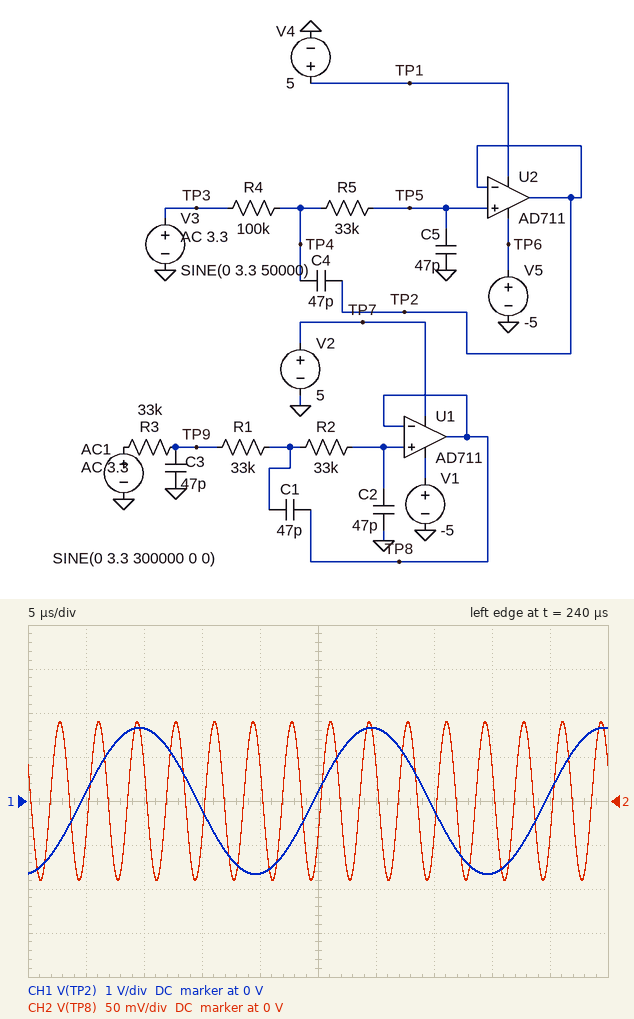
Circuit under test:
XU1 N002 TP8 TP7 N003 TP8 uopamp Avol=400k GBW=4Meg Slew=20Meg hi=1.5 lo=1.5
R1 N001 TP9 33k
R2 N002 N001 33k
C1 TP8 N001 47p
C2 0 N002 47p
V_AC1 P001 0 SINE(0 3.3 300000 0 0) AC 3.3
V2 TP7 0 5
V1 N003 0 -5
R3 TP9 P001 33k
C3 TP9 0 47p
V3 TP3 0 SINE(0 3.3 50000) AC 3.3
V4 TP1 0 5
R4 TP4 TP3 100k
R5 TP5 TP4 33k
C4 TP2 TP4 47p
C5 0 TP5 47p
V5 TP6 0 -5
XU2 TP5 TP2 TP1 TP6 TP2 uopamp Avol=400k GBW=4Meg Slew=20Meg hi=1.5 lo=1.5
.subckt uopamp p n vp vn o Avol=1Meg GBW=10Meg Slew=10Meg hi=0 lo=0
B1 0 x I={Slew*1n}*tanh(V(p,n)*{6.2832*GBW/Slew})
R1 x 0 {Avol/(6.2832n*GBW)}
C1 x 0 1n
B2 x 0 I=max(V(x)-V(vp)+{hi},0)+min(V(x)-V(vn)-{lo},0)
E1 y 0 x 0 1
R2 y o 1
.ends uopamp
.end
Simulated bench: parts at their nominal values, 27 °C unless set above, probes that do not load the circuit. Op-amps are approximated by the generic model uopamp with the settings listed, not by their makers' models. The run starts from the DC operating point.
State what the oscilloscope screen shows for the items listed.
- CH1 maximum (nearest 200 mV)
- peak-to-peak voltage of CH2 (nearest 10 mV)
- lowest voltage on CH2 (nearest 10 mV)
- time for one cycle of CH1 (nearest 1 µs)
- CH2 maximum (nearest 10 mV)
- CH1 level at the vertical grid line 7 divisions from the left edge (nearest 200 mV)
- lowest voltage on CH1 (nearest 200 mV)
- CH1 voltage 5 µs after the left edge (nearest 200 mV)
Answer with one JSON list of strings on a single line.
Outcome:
["1.6 V", "180 mV", "-90 mV", "20 µs", "90 mV", "-200 mV", "-1.6 V", "200 mV"]
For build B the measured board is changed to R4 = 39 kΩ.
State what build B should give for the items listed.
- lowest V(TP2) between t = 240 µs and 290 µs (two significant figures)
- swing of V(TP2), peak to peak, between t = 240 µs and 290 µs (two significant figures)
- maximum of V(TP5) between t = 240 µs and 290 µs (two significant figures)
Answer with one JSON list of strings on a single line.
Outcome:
["-2.6 V", "5.2 V", "2.6 V"]
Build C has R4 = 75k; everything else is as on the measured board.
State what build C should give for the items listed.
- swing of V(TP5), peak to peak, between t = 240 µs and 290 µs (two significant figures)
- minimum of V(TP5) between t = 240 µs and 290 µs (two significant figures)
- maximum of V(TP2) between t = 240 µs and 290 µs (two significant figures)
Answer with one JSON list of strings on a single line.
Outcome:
["4.0 V", "-2.0 V", "2.0 V"]
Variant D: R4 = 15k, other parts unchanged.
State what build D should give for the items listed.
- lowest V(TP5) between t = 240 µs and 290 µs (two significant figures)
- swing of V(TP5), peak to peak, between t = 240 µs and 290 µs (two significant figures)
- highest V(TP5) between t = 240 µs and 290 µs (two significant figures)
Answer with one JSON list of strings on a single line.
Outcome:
["-2.9 V", "5.8 V", "2.9 V"]
